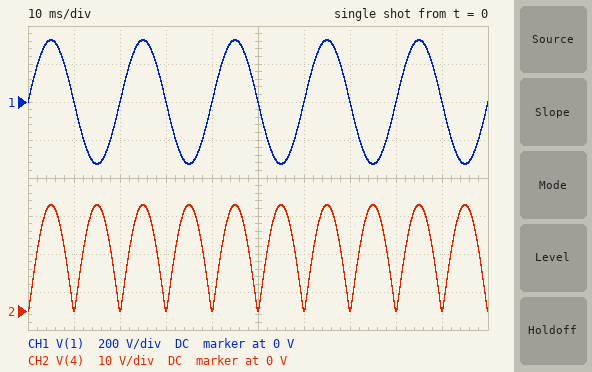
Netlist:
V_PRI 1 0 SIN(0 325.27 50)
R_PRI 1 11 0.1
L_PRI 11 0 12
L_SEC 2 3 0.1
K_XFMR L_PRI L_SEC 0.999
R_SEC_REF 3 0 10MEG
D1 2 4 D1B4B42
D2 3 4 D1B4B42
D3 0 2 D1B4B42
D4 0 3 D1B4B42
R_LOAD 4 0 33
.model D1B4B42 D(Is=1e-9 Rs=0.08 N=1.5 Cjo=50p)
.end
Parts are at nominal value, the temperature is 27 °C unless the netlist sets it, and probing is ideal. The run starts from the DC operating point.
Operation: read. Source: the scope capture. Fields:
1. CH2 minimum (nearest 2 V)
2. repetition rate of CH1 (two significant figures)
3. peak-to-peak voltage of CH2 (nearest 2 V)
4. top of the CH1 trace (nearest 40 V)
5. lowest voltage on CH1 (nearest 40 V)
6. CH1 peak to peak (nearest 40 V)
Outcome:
0 V
50 Hz
28 V
320 V
-320 V
640 V
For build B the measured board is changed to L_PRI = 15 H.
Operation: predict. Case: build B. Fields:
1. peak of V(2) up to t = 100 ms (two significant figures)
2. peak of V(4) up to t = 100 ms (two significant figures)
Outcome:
26 V
25 V
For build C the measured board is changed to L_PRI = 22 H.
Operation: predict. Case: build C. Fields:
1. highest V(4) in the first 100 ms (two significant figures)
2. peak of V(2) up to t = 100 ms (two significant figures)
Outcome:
20 V
21 V
